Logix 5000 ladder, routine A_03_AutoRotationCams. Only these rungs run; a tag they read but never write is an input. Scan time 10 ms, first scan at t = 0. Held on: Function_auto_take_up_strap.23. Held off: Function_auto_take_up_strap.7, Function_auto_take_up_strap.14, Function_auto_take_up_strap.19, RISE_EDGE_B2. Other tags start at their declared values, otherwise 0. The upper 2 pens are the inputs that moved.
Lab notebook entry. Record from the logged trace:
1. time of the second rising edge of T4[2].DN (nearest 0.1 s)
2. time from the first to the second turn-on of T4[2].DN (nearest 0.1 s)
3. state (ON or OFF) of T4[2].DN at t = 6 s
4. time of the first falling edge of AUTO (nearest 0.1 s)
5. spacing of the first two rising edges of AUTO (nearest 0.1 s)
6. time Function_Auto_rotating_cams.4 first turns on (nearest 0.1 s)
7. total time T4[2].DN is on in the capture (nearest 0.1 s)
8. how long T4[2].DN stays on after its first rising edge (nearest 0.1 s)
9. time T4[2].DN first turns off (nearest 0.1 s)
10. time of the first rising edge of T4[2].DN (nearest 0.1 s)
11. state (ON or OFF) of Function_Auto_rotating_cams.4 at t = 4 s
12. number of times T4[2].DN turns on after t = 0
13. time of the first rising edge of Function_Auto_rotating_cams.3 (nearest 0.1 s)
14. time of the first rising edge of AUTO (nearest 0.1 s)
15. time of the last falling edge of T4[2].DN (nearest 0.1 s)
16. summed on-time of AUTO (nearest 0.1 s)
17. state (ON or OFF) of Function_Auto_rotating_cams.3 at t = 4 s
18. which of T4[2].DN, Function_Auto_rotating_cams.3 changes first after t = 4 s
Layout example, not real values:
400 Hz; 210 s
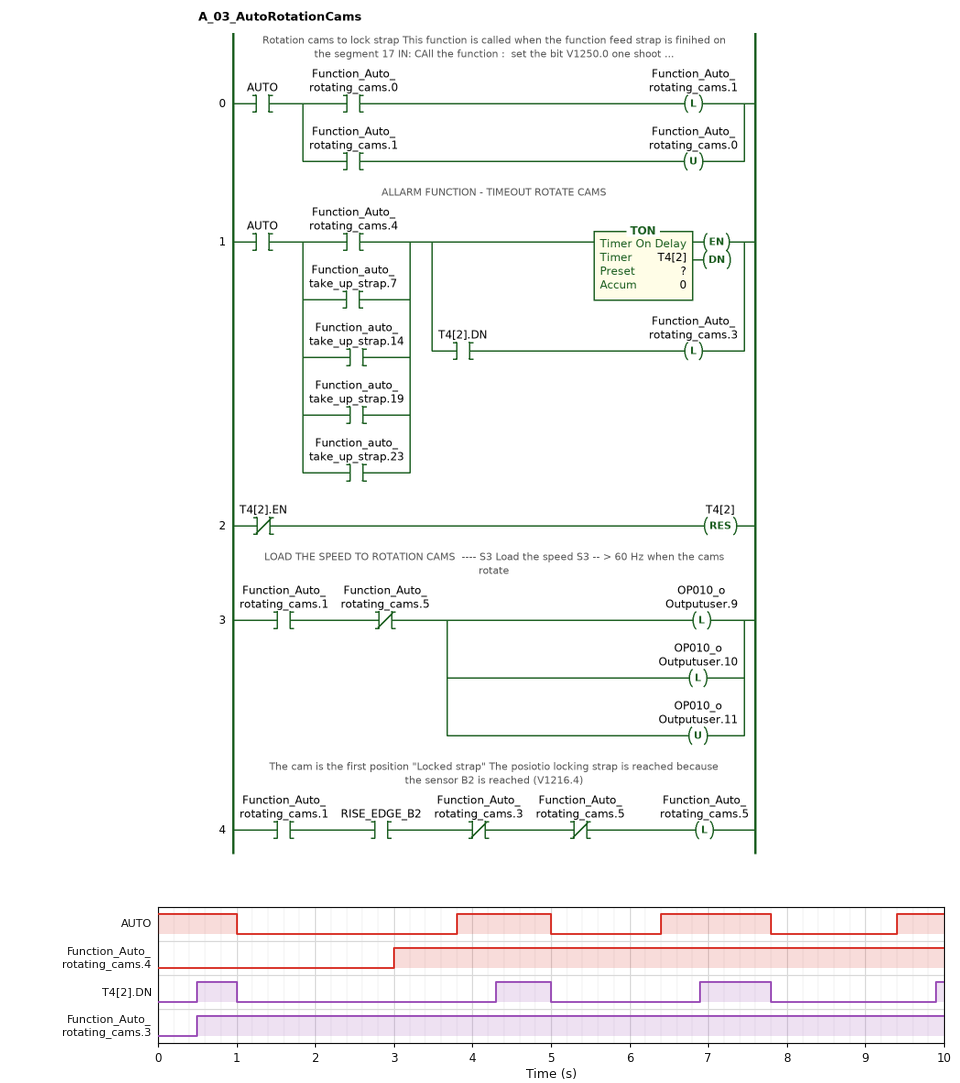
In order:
4.3 s; 3.8 s; OFF; 1.0 s; 2.6 s; 3.0 s; 2.2 s; 0.5 s; 1.0 s; 0.5 s; ON; 4; 0.5 s; 3.8 s; 7.8 s; 4.2 s; ON; T4[2].DN
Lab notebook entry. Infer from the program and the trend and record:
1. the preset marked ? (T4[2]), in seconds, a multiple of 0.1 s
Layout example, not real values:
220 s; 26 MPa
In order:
0.5 s
